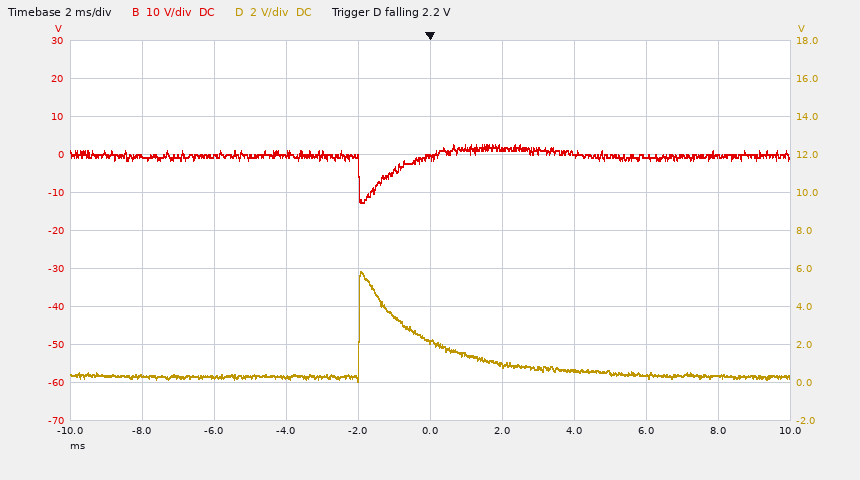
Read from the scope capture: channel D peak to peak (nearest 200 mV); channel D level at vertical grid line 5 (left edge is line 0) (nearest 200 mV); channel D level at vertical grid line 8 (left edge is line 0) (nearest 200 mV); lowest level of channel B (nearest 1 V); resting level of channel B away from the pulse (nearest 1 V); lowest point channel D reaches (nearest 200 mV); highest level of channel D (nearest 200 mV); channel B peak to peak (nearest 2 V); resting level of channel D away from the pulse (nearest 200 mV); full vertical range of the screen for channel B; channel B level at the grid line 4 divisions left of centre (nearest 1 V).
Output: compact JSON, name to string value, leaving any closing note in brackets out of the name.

{"channel D peak to peak": "5.8 V", "channel D level at vertical grid line 5 (left edge is line 0)": "2.2 V", "channel D level at vertical grid line 8 (left edge is line 0)": "400 mV", "lowest level of channel B": "-13 V", "resting level of channel B away from the pulse": "0 V", "lowest point channel D reaches": "0.0 V", "highest level of channel D": "5.8 V", "channel B peak to peak": "16 V", "resting level of channel D away from the pulse": "400 mV", "full vertical range of the screen for channel B": "100 V", "channel B level at the grid line 4 divisions left of centre": "0 V"}
